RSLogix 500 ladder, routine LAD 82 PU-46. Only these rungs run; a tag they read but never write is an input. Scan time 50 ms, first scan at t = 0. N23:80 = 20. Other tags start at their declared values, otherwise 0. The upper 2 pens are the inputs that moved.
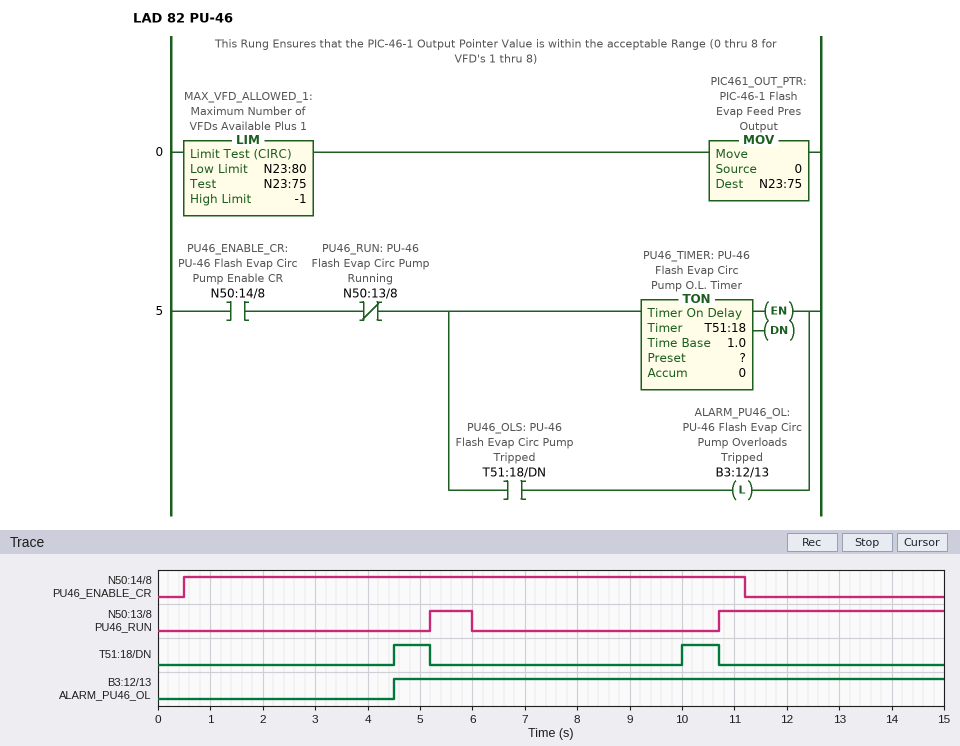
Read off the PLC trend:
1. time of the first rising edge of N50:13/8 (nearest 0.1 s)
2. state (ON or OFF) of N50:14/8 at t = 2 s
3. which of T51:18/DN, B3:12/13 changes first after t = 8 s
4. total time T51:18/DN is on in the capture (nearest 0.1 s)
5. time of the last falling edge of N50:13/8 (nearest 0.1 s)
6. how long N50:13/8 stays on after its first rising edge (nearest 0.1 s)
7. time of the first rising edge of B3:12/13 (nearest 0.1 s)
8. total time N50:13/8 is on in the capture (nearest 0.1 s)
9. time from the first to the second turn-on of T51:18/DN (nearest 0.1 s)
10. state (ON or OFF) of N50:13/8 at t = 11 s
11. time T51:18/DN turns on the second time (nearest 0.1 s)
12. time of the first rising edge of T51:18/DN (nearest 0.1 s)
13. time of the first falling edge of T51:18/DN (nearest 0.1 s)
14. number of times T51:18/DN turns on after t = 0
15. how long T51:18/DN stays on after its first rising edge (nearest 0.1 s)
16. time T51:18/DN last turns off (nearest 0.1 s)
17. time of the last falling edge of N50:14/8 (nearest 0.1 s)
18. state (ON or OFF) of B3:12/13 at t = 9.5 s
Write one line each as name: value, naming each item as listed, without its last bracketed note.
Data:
time of the first rising edge of N50:13/8: 5.2 s
state (ON or OFF) of N50:14/8 at t = 2 s: ON
which of T51:18/DN, B3:12/13 changes first after t = 8 s: T51:18/DN
total time T51:18/DN is on in the capture: 1.4 s
time of the last falling edge of N50:13/8: 6.0 s
how long N50:13/8 stays on after its first rising edge: 0.8 s
time of the first rising edge of B3:12/13: 4.5 s
total time N50:13/8 is on in the capture: 5.1 s
time from the first to the second turn-on of T51:18/DN: 5.5 s
state (ON or OFF) of N50:13/8 at t = 11 s: ON
time T51:18/DN turns on the second time: 10.0 s
time of the first rising edge of T51:18/DN: 4.5 s
time of the first falling edge of T51:18/DN: 5.2 s
number of times T51:18/DN turns on after t = 0: 2
how long T51:18/DN stays on after its first rising edge: 0.7 s
time T51:18/DN last turns off: 10.7 s
time of the last falling edge of N50:14/8: 11.2 s
state (ON or OFF) of B3:12/13 at t = 9.5 s: ON
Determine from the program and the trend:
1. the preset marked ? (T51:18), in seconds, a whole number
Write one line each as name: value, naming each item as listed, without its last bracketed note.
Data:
the preset marked ? (T51:18), in seconds, a whole number: 4 s
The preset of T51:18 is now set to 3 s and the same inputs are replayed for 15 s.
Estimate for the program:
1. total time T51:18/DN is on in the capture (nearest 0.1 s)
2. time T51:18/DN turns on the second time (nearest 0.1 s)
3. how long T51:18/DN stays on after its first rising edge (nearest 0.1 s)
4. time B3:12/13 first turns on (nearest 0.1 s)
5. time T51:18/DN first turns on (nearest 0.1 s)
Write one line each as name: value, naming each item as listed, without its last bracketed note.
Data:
total time T51:18/DN is on in the capture: 3.4 s
time T51:18/DN turns on the second time: 9.0 s
how long T51:18/DN stays on after its first rising edge: 1.7 s
time B3:12/13 first turns on: 3.5 s
time T51:18/DN first turns on: 3.5 s
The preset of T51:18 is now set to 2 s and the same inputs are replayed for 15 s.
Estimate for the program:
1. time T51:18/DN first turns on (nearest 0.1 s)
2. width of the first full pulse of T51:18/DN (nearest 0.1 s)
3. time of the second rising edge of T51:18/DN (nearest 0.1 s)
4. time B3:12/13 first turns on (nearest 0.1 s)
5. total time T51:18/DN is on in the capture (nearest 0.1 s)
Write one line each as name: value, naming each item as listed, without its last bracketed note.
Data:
time T51:18/DN first turns on: 2.5 s
width of the first full pulse of T51:18/DN: 2.7 s
time of the second rising edge of T51:18/DN: 8.0 s
time B3:12/13 first turns on: 2.5 s
total time T51:18/DN is on in the capture: 5.4 s
